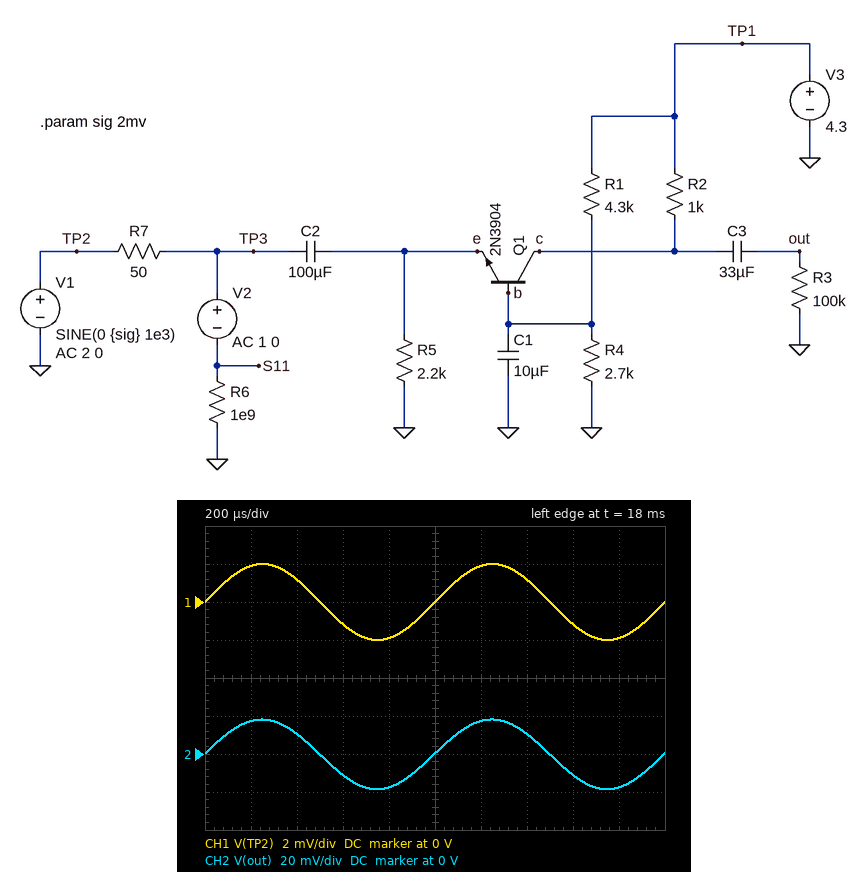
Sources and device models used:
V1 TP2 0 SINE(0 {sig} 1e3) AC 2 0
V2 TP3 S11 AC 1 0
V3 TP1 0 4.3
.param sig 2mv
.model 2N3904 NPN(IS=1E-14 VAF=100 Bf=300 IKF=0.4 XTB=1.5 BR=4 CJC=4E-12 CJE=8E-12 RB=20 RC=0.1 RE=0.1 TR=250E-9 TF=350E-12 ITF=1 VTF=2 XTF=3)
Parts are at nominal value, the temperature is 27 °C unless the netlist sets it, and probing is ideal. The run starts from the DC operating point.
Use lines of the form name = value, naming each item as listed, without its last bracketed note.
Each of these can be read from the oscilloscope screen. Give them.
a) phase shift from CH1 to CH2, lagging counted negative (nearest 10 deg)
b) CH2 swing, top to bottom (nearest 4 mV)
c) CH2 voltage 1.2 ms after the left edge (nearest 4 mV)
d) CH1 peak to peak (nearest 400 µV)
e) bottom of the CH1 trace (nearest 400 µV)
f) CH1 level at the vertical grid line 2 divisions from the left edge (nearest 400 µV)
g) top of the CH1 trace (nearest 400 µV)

phase shift from CH1 to CH2, lagging counted negative = 0 deg
CH2 swing, top to bottom = 36 mV
CH2 voltage 1.2 ms after the left edge = 16 mV
CH1 peak to peak = 4.0 mV
bottom of the CH1 trace = -2.0 mV
CH1 level at the vertical grid line 2 divisions from the left edge = 1.2 mV
top of the CH1 trace = 2.0 mV
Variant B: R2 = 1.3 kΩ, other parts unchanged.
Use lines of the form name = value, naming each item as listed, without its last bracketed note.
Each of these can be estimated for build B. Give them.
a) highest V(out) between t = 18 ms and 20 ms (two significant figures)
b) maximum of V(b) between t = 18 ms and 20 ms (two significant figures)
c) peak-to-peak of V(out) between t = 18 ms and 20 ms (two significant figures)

highest V(out) between t = 18 ms and 20 ms = 24 mV
maximum of V(b) between t = 18 ms and 20 ms = 1.7 V
peak-to-peak of V(out) between t = 18 ms and 20 ms = 48 mV
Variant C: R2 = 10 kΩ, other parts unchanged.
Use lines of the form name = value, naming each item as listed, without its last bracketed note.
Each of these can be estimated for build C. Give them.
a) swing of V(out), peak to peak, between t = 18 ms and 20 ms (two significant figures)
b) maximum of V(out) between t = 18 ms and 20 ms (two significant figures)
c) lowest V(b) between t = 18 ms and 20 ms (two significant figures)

swing of V(out), peak to peak, between t = 18 ms and 20 ms = 6.0 mV
maximum of V(out) between t = 18 ms and 20 ms = 3.1 mV
lowest V(b) between t = 18 ms and 20 ms = 1.5 V
